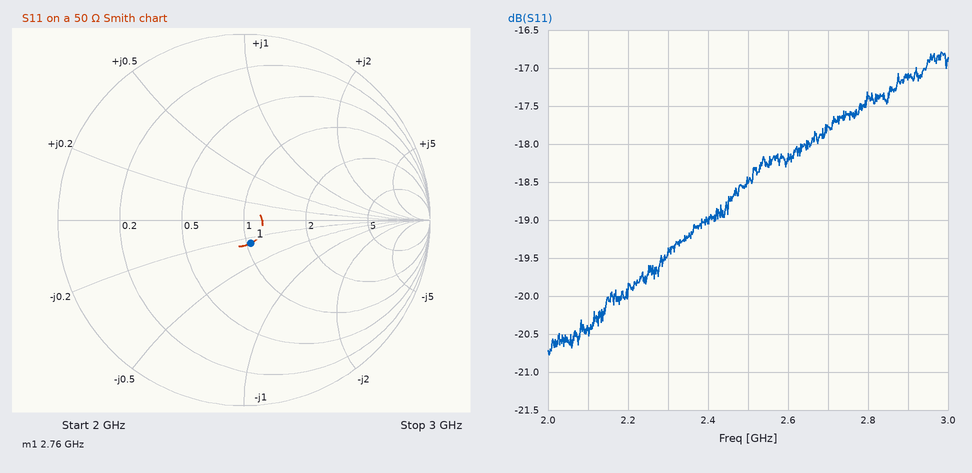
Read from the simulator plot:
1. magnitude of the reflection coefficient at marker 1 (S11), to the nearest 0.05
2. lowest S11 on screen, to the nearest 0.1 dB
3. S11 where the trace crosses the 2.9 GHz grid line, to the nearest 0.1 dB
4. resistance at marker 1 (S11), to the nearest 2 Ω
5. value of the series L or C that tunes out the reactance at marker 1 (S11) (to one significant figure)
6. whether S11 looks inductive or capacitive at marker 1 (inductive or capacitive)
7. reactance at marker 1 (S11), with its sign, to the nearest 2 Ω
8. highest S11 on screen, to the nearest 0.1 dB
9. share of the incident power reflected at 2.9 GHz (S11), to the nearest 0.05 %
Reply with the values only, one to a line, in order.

0.15
-20.8 dB
-17.1 dB
52 Ω
800 pH
capacitive
-14 Ω
-16.8 dB
1.95 %
